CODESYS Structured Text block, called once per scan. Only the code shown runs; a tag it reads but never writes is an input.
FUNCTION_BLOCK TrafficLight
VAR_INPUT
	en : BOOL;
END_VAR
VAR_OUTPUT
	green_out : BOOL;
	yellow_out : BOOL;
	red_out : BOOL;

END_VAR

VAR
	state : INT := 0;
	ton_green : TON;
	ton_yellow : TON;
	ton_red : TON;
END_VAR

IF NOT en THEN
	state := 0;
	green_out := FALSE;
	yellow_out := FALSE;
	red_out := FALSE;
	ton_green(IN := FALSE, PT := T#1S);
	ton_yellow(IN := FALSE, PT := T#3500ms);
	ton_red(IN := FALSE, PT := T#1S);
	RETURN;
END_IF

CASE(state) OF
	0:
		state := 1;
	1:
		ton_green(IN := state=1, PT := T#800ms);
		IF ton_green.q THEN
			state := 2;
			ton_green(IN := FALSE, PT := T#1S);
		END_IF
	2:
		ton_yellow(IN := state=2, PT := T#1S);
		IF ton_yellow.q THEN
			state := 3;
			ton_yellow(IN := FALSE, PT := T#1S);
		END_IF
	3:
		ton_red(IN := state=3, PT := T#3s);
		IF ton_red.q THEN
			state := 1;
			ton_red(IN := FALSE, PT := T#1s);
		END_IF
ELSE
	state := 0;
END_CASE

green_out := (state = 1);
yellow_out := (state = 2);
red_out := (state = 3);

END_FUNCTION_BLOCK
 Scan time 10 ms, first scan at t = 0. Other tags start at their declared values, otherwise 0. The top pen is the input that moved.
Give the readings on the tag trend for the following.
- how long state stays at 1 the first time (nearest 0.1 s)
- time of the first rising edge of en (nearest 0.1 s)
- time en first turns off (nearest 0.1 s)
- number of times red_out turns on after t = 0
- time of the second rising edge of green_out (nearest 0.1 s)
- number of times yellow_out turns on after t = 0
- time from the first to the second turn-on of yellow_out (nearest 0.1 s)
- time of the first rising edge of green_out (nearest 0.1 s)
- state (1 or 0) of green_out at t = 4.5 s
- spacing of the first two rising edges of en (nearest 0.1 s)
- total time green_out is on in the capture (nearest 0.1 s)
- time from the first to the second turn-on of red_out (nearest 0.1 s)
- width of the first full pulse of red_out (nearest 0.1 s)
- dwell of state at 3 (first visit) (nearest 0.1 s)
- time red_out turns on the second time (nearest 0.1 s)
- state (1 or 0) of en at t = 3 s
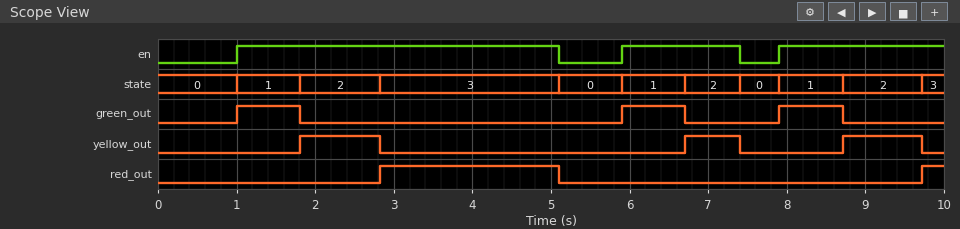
0.8 s
1.0 s
5.1 s
2
5.9 s
3
4.9 s
1.0 s
0
4.9 s
2.4 s
6.9 s
2.3 s
2.3 s
9.7 s
1
